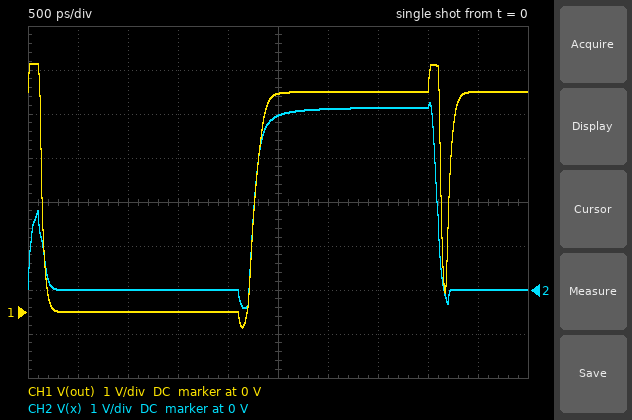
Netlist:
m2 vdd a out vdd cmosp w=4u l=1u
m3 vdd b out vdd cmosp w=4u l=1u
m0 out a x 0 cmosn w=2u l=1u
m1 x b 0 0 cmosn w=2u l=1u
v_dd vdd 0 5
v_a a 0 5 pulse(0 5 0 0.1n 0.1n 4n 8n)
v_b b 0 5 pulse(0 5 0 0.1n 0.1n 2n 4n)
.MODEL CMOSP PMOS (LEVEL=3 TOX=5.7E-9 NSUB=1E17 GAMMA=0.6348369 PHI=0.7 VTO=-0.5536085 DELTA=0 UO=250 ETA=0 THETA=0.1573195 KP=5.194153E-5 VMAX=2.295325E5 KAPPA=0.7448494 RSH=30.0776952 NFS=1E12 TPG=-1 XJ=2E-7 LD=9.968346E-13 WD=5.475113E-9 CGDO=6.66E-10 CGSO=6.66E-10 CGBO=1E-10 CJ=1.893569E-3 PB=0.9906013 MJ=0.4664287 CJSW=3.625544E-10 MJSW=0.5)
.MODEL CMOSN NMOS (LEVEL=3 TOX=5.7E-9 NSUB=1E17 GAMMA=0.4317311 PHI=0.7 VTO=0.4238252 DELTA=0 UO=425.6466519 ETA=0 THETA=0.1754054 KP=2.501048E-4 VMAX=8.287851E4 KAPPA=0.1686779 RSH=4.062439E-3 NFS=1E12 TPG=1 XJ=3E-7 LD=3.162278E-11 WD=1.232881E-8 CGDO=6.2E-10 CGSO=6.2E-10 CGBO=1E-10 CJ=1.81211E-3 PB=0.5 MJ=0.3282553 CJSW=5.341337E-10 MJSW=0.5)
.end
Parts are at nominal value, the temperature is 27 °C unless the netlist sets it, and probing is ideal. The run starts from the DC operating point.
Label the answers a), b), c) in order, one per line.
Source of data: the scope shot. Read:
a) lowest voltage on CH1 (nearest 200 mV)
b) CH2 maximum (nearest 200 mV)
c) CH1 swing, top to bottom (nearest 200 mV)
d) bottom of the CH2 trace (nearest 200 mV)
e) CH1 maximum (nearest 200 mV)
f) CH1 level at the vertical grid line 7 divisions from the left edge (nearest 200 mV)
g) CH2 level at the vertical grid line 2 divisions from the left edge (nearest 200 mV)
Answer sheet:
a) -400 mV
b) 4.2 V
c) 6.0 V
d) -400 mV
e) 5.6 V
f) 5.0 V
g) 0 V
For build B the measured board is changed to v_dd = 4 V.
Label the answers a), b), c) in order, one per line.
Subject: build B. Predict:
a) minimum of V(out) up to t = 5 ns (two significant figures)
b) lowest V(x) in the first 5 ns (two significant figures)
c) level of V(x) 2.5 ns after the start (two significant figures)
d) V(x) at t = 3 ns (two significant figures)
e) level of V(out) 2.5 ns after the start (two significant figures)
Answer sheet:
a) -600 mV
b) -590 mV
c) 3.7 V
d) 4.0 V
e) 3.8 V
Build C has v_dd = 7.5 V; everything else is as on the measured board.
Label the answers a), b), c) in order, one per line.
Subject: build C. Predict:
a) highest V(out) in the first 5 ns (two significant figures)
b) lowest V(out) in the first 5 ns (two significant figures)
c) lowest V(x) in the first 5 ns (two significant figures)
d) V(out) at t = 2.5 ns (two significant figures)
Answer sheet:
a) 8.1 V
b) 850 mV
c) -320 mV
d) 7.5 V
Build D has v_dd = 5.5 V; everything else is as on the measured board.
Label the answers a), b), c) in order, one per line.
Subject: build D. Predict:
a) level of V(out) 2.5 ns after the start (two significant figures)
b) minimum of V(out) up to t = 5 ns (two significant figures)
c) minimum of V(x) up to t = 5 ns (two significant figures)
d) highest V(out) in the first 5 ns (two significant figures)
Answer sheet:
a) 5.5 V
b) -280 mV
c) -340 mV
d) 6.1 V
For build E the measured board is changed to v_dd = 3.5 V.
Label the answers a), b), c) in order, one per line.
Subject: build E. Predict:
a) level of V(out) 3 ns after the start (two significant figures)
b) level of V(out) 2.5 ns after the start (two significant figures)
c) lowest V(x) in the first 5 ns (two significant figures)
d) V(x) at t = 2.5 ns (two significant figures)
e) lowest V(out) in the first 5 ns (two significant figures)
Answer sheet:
a) 3.5 V
b) 3.3 V
c) -600 mV
d) 3.2 V
e) -620 mV
